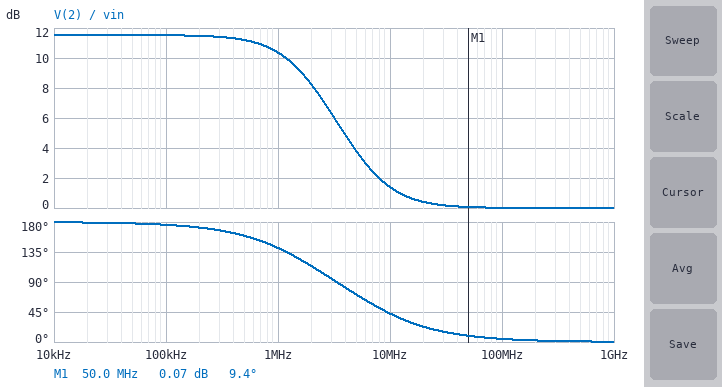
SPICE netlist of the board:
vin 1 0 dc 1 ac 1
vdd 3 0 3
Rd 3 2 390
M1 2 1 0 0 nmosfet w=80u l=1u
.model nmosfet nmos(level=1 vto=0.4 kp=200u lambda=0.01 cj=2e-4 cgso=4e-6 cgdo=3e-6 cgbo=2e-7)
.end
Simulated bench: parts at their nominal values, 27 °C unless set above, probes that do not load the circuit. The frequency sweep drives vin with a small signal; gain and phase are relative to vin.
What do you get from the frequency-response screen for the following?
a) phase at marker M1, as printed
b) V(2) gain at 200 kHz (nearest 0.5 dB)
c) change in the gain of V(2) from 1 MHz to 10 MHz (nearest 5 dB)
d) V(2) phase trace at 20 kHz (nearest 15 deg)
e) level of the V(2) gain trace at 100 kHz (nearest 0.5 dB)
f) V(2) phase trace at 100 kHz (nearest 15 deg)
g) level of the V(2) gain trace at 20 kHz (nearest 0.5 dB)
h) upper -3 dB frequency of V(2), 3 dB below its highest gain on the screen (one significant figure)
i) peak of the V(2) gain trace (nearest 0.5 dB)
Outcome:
9.4 deg
11.5 dB
-10 dB
180 deg
11.5 dB
180 deg
11.5 dB
2 MHz
11.5 dB
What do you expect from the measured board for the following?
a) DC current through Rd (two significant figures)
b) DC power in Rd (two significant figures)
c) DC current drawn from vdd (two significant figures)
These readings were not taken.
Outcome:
2.9 mA
3.4 mW
2.9 mA
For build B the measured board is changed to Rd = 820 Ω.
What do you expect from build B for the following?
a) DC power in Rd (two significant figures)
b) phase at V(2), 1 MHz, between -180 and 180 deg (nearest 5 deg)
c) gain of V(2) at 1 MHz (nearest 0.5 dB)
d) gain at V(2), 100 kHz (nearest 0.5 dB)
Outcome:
6.9 mW
120 deg
14.0 dB
17.5 dB
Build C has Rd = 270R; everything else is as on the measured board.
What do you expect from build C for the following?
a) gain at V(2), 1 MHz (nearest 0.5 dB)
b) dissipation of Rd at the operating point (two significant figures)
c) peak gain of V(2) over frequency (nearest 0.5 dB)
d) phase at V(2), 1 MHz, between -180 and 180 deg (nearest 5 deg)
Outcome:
8.0 dB
2.3 mW
8.5 dB
150 deg
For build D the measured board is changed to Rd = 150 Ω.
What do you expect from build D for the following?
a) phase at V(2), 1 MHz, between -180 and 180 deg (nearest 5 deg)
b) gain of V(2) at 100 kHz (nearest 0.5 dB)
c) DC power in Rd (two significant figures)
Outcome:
160 deg
3.5 dB
1.3 mW
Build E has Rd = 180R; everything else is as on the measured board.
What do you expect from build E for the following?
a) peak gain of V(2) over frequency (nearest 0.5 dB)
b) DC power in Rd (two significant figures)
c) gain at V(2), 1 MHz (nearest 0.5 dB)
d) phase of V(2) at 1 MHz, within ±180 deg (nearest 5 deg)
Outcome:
5.0 dB
1.6 mW
4.5 dB
155 deg
